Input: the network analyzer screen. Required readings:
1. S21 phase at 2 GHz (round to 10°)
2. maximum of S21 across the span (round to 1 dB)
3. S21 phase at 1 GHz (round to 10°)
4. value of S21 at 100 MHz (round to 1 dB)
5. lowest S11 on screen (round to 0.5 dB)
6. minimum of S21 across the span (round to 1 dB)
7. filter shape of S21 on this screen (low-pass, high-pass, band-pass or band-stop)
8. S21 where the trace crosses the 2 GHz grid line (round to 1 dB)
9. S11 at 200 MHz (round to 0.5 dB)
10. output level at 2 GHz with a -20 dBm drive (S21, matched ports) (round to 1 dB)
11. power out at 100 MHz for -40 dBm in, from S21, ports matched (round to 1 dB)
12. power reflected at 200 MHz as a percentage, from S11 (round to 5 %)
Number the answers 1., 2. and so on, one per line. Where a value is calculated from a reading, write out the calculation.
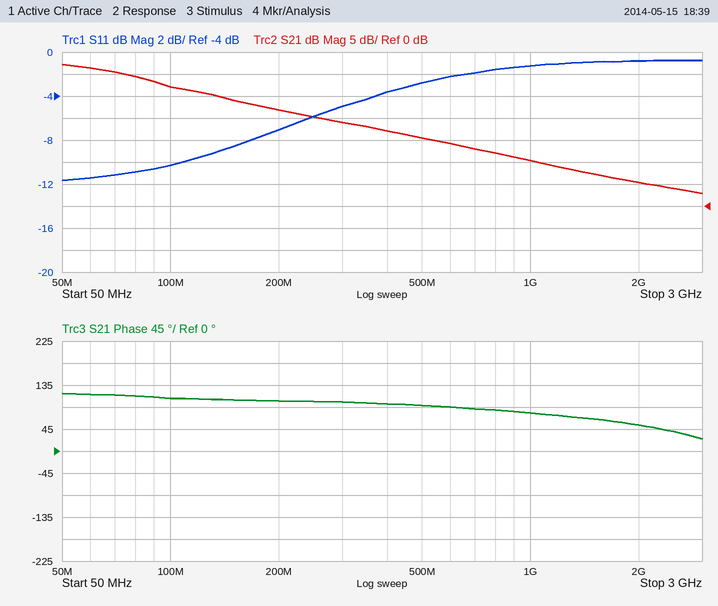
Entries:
1. 50°
2. 32 dB
3. 80°
4. 27 dB
5. -11.5 dB
6. 3 dB
7. low-pass
8. 5 dB
9. -7.0 dB
10. -20 dBm + (5 dB) = -15 dBm
11. -40 dBm + (27 dB) = -13 dBm
12. 10^(-7/10) ≈ 20 %
